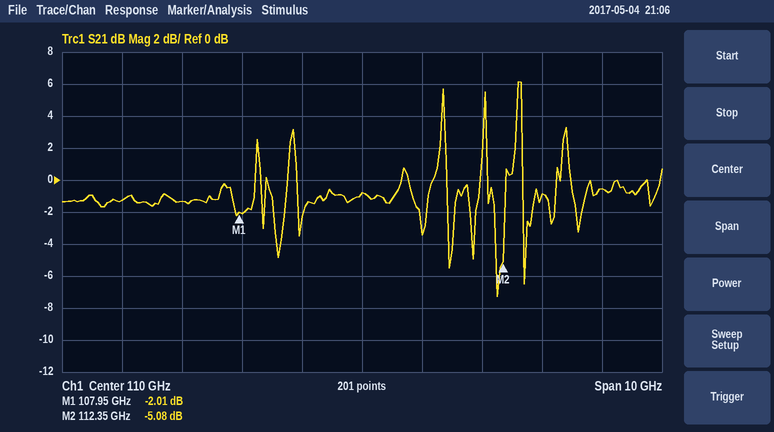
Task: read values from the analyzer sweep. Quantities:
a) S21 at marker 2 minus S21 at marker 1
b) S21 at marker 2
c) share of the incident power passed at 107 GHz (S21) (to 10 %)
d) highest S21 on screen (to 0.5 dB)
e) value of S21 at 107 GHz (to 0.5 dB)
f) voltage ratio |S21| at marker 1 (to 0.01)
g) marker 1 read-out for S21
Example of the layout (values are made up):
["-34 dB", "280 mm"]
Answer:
["-3.07 dB", "-5.08 dB", "70 %", "6.0 dB", "-1.5 dB", "0.79", "-2.01 dB"]
